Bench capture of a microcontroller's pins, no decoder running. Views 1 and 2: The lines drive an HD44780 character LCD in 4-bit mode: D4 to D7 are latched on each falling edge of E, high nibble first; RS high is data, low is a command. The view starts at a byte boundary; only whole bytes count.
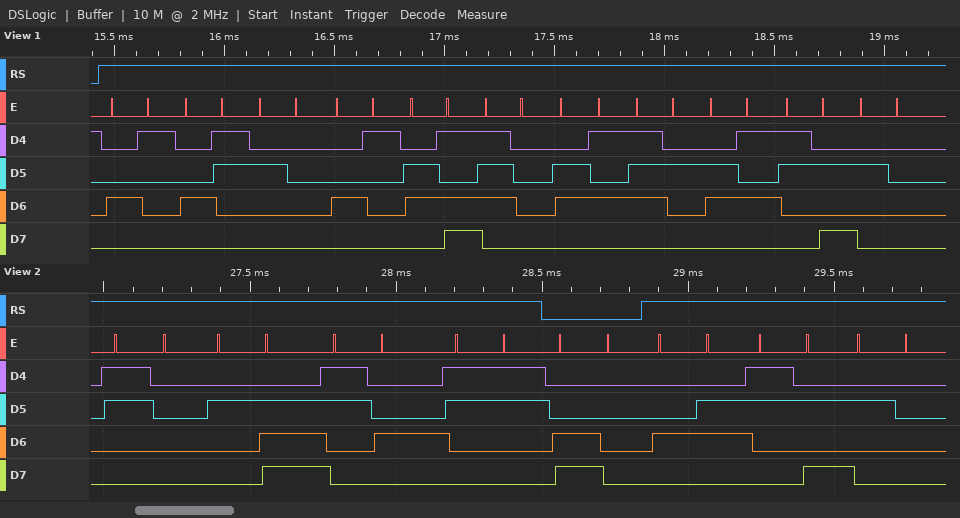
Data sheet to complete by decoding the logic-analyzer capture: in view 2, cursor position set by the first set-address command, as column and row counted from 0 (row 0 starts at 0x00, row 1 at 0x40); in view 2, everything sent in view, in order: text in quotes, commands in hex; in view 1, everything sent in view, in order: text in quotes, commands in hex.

column 0, row 1
"0.43" 0xC0 "F: "
"AC Ampere: "
